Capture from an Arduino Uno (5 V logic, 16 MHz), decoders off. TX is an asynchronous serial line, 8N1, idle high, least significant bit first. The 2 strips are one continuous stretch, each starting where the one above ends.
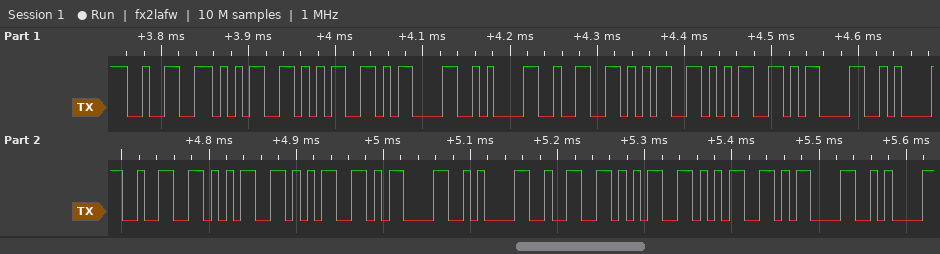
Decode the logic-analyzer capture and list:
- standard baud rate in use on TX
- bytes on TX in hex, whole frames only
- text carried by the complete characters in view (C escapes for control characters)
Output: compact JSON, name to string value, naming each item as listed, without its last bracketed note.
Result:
{"standard baud rate in use on TX": "115200 baud", "bytes on TX in hex, whole frames only": "32 35 35 0D 0A 32 35 35 0D 0A 32 35 35 0D 0A 32 35 35 0D 0A", "text carried by the complete characters in view": "\"255\\r\\n255\\r\\n255\\r\\n255\\r\\n\""}
